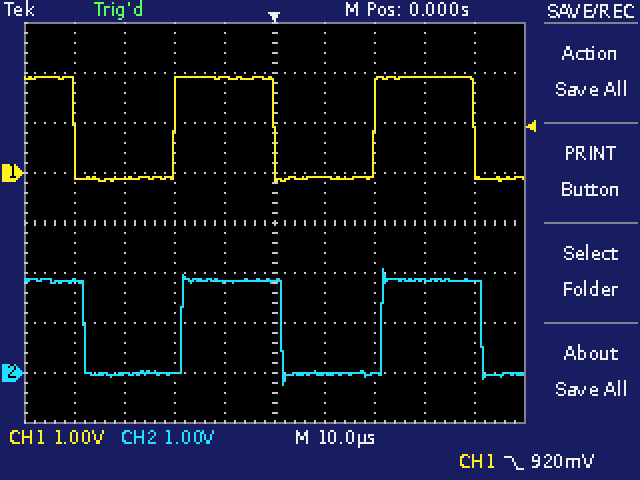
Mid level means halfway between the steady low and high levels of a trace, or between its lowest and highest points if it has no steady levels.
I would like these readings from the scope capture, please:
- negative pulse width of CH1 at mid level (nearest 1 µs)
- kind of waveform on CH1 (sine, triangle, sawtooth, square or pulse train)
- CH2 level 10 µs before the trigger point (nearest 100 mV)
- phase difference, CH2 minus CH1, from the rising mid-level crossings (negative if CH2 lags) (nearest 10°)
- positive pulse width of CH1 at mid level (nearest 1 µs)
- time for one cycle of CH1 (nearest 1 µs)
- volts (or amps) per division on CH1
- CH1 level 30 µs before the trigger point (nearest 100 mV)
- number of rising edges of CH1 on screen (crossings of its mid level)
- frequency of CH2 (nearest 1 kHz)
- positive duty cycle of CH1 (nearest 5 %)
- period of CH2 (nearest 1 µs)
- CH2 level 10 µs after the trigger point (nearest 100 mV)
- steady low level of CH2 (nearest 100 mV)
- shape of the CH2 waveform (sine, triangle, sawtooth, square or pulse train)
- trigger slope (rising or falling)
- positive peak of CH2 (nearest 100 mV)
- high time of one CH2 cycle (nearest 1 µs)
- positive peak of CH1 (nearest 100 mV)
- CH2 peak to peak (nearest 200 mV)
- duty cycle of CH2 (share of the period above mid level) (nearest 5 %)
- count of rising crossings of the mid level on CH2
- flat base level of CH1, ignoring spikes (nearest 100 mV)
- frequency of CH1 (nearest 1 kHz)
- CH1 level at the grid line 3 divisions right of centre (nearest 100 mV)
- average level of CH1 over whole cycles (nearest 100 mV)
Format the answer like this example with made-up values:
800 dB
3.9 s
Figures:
20 µs
square
1.8 V
-10°
20 µs
40 µs
1 V
-100 mV
2
25 kHz
50 %
40 µs
0.0 V
0.0 V
square
falling
2.1 V
20 µs
1.9 V
2.4 V
50 %
2
-100 mV
25 kHz
1.9 V
900 mV
